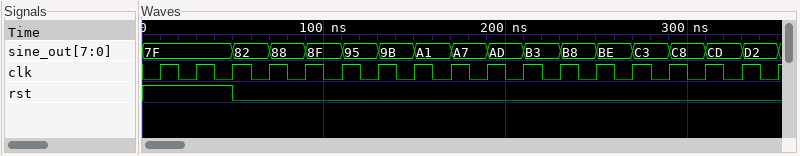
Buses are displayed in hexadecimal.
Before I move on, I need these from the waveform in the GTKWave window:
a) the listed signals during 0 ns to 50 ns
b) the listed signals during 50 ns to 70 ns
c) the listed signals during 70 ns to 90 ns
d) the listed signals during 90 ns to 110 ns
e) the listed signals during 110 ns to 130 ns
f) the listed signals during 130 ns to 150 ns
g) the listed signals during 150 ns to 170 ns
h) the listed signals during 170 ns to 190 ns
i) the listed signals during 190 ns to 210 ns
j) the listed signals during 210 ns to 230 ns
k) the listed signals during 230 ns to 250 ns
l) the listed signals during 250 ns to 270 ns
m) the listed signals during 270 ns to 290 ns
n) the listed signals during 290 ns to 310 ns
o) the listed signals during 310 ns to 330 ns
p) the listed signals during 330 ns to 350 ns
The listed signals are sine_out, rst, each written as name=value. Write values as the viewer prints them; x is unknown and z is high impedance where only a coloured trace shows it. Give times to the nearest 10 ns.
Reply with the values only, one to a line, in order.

sine_out=7F, rst=1
sine_out=82, rst=0
sine_out=88, rst=0
sine_out=8F, rst=0
sine_out=95, rst=0
sine_out=9B, rst=0
sine_out=A1, rst=0
sine_out=A7, rst=0
sine_out=AD, rst=0
sine_out=B3, rst=0
sine_out=B8, rst=0
sine_out=BE, rst=0
sine_out=C3, rst=0
sine_out=C8, rst=0
sine_out=CD, rst=0
sine_out=D2, rst=0
